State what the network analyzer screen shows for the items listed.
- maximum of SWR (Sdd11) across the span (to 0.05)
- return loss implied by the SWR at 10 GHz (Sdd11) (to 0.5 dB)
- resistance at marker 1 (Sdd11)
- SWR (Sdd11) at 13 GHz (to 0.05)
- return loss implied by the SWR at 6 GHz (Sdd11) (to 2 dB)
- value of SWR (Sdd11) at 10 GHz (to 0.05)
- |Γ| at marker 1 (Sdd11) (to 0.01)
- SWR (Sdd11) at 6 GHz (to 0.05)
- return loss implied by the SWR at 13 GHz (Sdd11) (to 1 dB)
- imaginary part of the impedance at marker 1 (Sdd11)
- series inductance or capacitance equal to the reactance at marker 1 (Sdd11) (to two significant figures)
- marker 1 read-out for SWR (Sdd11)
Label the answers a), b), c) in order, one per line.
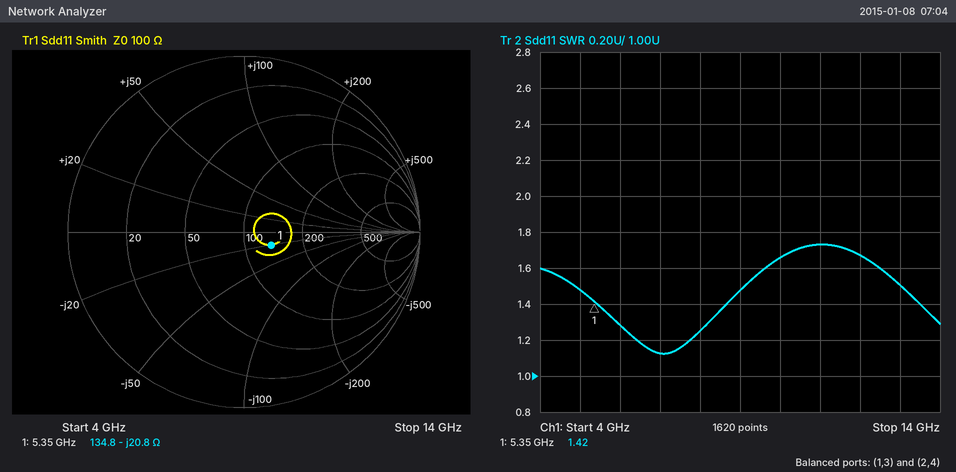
a) 1.75
b) 12.0 dB
c) 134.8 Ω
d) 1.50
e) 18 dB
f) 1.65
g) 0.17
h) 1.30
i) 14 dB
j) -20.8 Ω
k) 1.4 pF
l) 1.42
